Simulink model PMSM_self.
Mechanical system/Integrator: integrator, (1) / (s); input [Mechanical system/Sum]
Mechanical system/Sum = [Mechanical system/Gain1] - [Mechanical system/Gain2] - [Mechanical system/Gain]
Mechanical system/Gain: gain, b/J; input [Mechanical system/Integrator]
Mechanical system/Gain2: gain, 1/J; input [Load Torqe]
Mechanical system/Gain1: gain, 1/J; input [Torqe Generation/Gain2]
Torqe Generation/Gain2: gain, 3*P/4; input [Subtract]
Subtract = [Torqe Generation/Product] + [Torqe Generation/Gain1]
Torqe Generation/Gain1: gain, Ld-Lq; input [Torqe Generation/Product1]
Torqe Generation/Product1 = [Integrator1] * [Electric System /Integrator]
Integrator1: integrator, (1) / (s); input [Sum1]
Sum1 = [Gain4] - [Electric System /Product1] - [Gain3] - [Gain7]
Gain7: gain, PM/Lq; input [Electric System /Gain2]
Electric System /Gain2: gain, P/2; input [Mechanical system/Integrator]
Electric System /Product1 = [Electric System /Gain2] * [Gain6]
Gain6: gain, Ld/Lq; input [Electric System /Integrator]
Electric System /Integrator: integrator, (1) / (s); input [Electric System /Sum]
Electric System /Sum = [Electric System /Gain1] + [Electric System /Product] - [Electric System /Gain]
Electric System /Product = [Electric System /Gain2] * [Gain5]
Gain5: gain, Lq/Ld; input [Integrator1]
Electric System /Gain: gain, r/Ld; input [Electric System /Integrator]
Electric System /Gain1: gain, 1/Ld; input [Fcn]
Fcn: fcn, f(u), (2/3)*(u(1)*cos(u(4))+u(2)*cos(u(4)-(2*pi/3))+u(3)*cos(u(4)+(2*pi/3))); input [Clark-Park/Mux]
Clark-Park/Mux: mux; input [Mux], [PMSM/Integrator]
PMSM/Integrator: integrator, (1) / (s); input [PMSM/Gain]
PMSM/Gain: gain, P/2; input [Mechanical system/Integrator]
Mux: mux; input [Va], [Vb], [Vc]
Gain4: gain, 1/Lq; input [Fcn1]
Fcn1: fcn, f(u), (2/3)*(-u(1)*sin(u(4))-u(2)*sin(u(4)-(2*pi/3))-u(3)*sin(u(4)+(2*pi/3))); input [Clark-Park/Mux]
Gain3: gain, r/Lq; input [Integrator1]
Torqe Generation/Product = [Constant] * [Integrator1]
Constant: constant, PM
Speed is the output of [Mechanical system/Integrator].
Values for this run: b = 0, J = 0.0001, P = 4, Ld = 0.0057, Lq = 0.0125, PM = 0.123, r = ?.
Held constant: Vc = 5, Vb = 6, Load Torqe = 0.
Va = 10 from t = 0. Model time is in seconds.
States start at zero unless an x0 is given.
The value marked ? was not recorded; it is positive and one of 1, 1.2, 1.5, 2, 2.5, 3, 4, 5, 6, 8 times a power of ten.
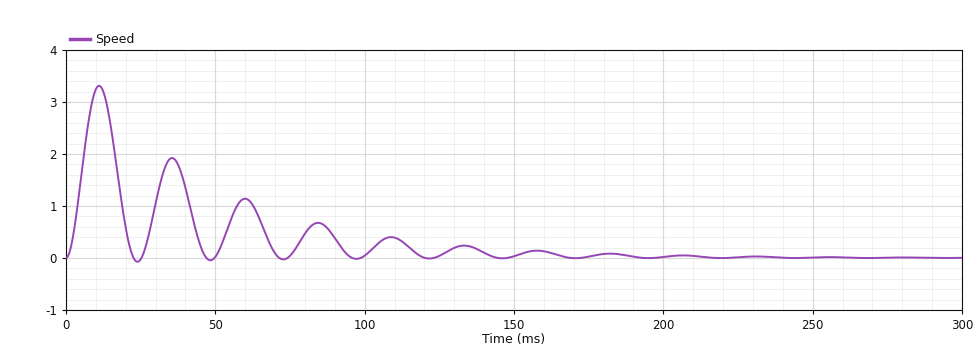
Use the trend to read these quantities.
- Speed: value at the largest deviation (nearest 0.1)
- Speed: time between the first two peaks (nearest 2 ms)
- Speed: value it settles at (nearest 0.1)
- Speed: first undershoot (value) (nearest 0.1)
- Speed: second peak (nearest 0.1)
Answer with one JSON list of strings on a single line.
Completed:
["3.3", "24 ms", "0.0", "-0.1", "1.9"]
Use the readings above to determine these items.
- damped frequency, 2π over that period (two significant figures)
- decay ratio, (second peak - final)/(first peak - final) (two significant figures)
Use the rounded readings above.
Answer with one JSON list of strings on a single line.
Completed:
["0.26 rad/ms", "0.58"]
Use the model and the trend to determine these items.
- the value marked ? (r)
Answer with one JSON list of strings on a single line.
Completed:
["0.8"]
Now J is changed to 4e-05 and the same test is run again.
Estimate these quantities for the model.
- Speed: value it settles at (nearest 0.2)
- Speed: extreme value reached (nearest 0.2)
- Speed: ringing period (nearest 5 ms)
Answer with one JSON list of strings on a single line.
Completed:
["0.0", "3.6", "15 ms"]
